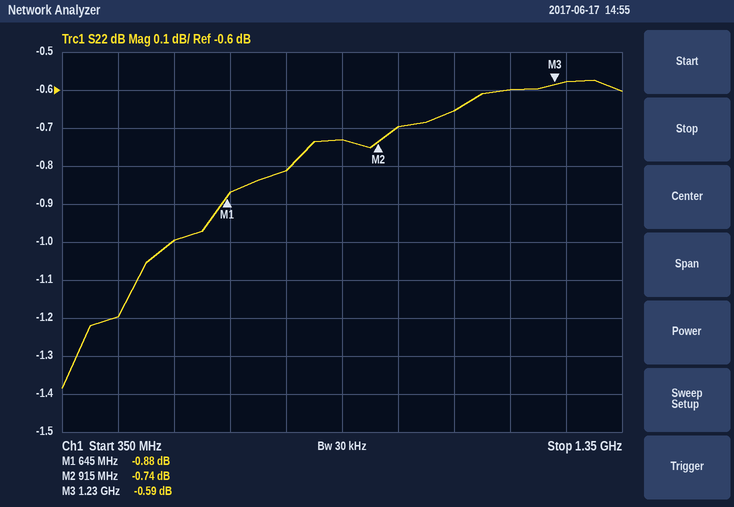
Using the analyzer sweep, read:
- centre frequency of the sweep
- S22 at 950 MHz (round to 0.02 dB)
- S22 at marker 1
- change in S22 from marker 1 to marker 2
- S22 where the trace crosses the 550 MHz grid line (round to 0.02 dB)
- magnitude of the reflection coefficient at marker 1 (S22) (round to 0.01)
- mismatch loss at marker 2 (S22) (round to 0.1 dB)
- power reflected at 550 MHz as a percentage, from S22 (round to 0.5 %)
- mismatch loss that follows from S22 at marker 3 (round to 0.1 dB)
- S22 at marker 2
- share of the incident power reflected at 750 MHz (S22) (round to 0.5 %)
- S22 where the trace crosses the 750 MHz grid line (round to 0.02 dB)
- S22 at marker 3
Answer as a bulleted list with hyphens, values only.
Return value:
- 850 MHz
- -0.70 dB
- -0.88 dB
- 0.14 dB
- -1.00 dB
- 0.90
- 8.1 dB
- 79.5 %
- 9.0 dB
- -0.74 dB
- 83.0 %
- -0.82 dB
- -0.59 dB
